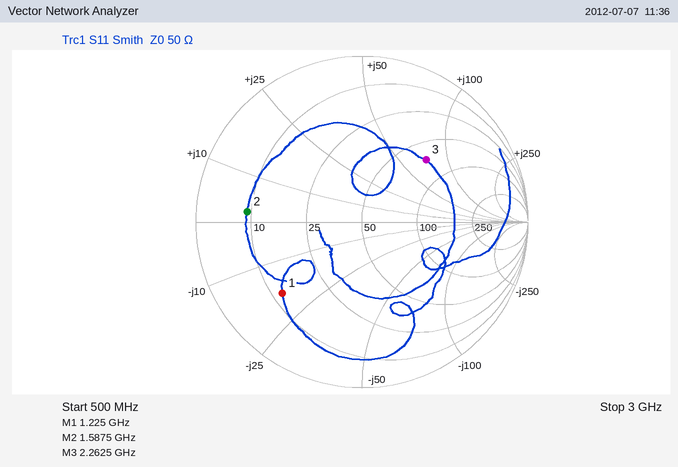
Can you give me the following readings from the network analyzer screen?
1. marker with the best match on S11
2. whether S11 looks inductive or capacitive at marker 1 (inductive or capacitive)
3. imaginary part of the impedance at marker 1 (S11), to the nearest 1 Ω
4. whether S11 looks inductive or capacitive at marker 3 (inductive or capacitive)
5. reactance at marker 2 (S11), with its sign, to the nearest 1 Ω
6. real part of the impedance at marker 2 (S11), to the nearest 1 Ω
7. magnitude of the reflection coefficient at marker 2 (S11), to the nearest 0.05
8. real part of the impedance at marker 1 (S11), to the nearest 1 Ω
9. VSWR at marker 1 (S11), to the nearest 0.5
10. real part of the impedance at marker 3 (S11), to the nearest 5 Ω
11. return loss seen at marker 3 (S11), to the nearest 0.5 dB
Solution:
marker 3
capacitive
-18 Ω
inductive
+2 Ω
9 Ω
0.70
12 Ω
4.5
70 Ω
5.5 dB
